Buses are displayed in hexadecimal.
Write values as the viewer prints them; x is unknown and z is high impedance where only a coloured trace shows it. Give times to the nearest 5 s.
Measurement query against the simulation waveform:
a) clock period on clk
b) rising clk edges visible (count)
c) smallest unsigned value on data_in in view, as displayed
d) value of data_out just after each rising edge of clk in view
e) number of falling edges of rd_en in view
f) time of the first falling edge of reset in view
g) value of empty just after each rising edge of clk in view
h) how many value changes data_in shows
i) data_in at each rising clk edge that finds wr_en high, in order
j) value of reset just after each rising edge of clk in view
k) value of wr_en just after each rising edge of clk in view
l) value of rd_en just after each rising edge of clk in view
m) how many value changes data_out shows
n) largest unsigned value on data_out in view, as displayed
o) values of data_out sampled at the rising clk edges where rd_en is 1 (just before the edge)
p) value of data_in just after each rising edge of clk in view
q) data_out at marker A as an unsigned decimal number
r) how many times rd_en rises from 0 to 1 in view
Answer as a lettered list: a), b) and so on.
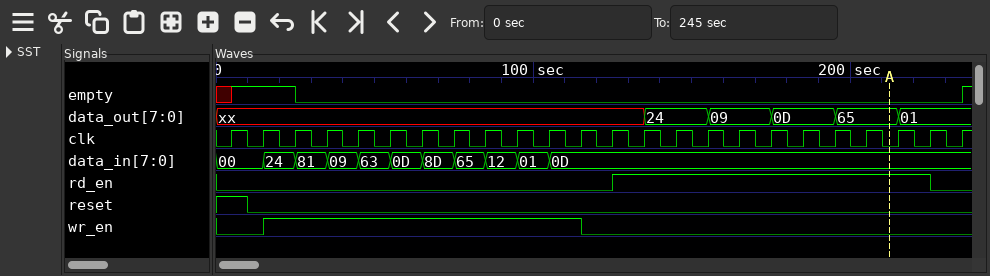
a) 10 s
b) 24
c) 00
d) xx, xx, xx, xx, xx, xx, xx, xx, xx, xx, xx, xx, xx, 24, 24, 09, 09, 0D, 0D, 65, 65, 01, 01, 01
e) 1
f) 10 s
g) 1 1 0 0 0 0 0 0 0 0 0 0 0 0 0 0 0 0 0 0 0 0 0 1
h) 10
i) 24, 81, 09, 63, 0D, 8D, 65, 12, 01, 0D
j) 1 0 0 0 0 0 0 0 0 0 0 0 0 0 0 0 0 0 0 0 0 0 0 0
k) 0 1 1 1 1 1 1 1 1 1 1 0 0 0 0 0 0 0 0 0 0 0 0 0
l) 0 0 0 0 0 0 0 0 0 0 0 0 1 1 1 1 1 1 1 1 1 1 0 0
m) 5
n) 65
o) xx, 24, 24, 09, 09, 0D, 0D, 65, 65, 01
p) 00, 24, 81, 09, 63, 0D, 8D, 65, 12, 01, 0D, 0D, 0D, 0D, 0D, 0D, 0D, 0D, 0D, 0D, 0D, 0D, 0D, 0D
q) 101
r) 1
